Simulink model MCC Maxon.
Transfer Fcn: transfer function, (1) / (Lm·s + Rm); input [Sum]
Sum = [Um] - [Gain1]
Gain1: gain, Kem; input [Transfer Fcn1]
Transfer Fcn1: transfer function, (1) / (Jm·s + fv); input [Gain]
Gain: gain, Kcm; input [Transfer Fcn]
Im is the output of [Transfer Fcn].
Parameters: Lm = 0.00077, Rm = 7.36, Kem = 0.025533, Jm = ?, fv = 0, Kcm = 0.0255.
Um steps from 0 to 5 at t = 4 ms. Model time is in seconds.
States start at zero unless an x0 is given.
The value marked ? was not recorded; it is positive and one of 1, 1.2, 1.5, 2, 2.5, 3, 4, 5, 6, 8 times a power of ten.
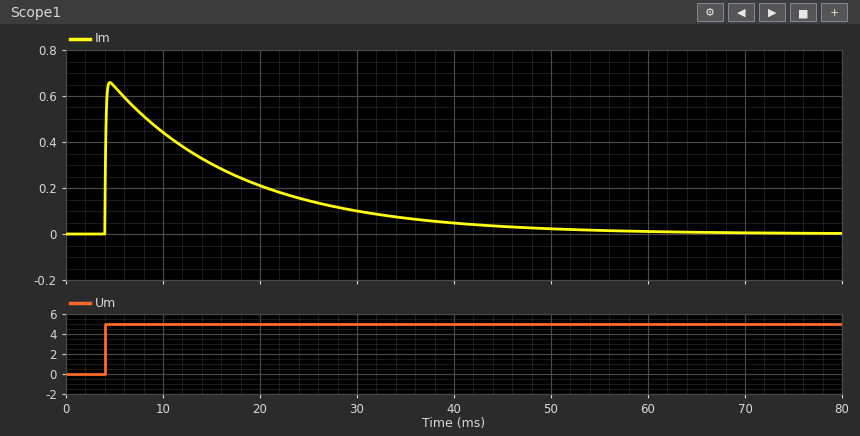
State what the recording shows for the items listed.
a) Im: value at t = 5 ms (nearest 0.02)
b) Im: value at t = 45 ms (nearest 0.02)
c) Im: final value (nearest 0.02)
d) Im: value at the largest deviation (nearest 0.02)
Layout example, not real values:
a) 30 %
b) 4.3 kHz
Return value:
a) 0.64
b) 0.04
c) 0.00
d) 0.66
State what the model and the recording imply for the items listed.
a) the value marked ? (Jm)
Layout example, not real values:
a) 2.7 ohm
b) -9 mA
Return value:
a) 1.2e-06
